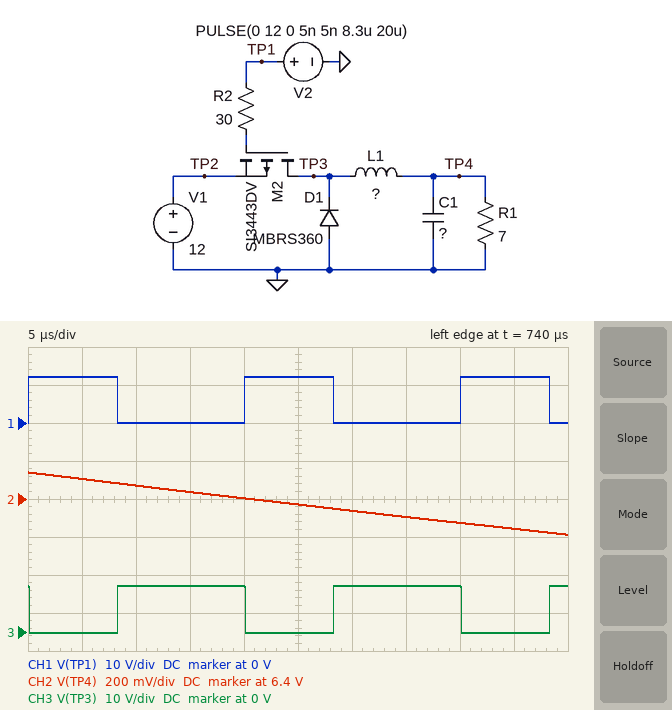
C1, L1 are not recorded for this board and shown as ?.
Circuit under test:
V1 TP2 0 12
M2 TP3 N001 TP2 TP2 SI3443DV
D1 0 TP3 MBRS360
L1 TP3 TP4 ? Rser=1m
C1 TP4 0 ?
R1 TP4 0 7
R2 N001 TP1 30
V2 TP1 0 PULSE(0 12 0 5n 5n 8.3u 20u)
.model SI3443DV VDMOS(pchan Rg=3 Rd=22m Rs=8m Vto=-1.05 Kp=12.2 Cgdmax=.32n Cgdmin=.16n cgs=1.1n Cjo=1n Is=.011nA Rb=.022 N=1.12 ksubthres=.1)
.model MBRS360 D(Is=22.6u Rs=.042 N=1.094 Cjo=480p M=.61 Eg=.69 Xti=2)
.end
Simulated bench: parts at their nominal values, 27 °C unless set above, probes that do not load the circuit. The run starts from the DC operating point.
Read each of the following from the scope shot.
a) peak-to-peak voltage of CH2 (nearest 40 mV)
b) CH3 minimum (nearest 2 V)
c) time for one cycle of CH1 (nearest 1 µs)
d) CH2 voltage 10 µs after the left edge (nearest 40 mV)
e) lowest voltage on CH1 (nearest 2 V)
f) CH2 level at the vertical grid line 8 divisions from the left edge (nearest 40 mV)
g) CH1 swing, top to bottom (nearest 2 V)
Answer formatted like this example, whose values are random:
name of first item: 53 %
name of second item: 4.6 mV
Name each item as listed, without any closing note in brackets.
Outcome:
peak-to-peak voltage of CH2: 320 mV
CH3 minimum: 0 V
time for one cycle of CH1: 20 µs
CH2 voltage 10 µs after the left edge: 6.48 V
lowest voltage on CH1: 0 V
CH2 level at the vertical grid line 8 divisions from the left edge: 6.28 V
CH1 swing, top to bottom: 12 V
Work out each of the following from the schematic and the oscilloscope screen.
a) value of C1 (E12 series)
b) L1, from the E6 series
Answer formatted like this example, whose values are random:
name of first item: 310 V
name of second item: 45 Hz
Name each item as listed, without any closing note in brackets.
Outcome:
value of C1: 82 µF
L1, from the E6 series: 1.5 mH
